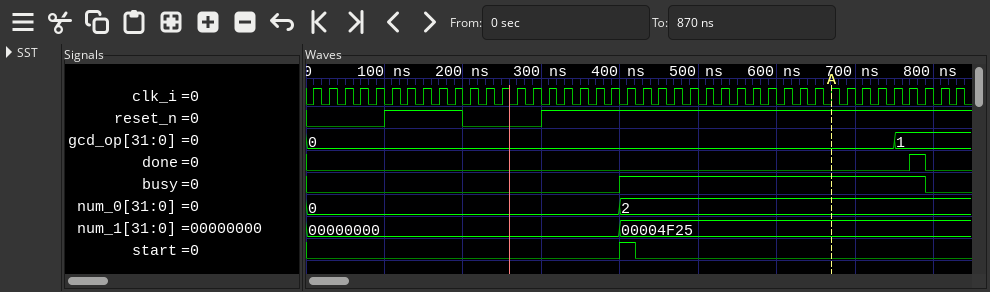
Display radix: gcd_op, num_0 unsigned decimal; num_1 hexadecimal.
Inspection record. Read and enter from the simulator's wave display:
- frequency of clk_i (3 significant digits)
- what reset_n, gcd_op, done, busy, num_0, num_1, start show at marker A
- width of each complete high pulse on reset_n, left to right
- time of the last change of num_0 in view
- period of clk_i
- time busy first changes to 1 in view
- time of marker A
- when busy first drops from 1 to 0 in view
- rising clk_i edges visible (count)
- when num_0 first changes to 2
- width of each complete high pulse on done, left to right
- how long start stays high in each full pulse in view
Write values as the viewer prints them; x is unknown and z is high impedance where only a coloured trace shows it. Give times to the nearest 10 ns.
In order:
50.0 MHz
reset_n=1, gcd_op=0, done=0, busy=1, num_0=2, num_1=00004F25, start=0
100 ns
400 ns
20 ns
400 ns
670 ns
790 ns
42
400 ns
20 ns
20 ns
